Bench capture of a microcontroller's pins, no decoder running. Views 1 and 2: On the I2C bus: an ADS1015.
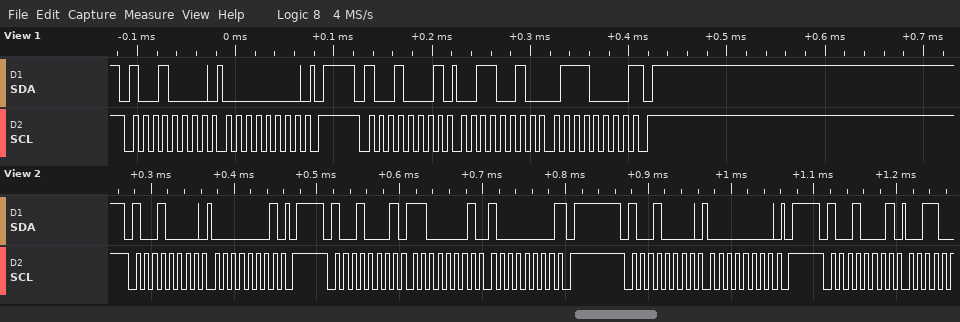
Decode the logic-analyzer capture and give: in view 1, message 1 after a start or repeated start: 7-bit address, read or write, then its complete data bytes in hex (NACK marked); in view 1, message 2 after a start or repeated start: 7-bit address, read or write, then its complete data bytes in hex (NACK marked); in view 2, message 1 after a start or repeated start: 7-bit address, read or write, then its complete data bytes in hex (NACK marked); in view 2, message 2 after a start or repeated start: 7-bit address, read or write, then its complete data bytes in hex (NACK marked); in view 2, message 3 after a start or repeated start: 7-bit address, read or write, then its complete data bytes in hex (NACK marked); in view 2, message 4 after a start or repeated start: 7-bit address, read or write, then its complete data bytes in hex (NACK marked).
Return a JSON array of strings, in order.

["0x48 write: 00", "0x48 read: 32 70 NACK", "0x48 write: 01", "0x48 read: C1 80 NACK", "0x48 write: 00", "0x48 read"]
